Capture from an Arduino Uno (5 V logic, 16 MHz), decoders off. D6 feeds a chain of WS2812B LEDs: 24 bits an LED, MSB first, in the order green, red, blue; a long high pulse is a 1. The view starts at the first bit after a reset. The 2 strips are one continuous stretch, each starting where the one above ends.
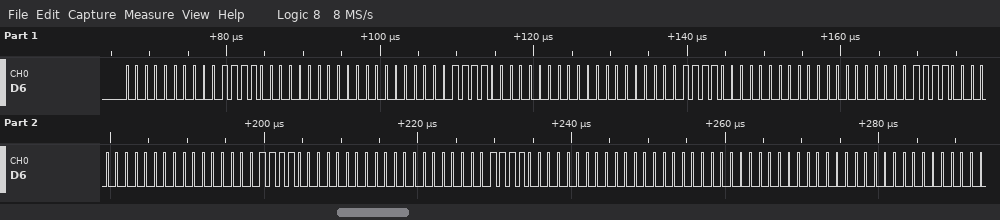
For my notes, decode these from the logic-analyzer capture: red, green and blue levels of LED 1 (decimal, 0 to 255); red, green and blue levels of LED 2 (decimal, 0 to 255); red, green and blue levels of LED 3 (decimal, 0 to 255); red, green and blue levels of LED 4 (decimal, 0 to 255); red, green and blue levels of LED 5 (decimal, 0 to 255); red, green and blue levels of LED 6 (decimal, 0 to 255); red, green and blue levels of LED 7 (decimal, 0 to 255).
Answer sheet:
60, 0, 0
60, 0, 0
60, 0, 0
60, 0, 0
60, 0, 0
60, 0, 0
0, 0, 0
